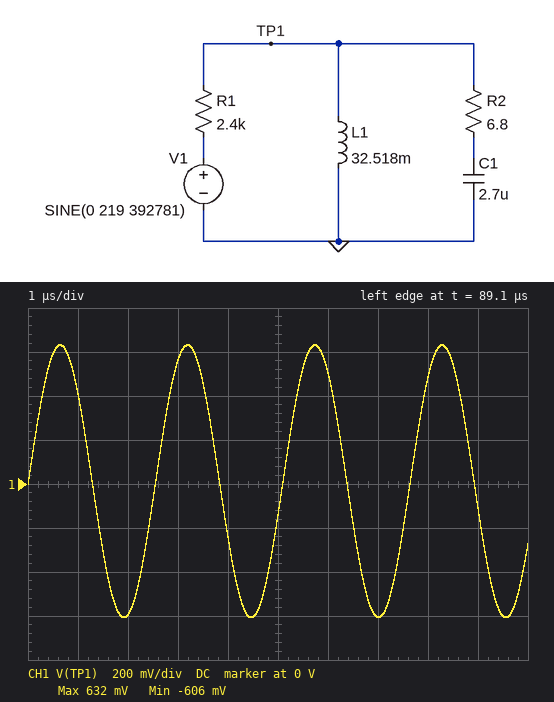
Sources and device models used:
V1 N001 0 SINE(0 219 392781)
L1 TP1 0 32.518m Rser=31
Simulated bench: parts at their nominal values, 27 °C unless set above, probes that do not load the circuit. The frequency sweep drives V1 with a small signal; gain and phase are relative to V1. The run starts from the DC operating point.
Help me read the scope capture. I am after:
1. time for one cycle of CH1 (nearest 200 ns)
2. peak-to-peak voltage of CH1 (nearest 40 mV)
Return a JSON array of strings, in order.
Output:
["2.6 µs", "1.24 V"]
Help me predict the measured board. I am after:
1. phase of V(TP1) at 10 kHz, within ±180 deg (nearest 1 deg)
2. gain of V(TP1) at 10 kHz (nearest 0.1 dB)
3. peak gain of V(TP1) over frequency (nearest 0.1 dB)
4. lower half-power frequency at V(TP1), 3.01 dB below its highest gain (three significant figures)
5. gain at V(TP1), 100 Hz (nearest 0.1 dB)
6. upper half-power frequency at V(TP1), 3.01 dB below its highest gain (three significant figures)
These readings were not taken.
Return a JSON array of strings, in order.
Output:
["-41 deg", "-48.5 dB", "-18.3 dB", "442 Hz", "-36.0 dB", "652 Hz"]
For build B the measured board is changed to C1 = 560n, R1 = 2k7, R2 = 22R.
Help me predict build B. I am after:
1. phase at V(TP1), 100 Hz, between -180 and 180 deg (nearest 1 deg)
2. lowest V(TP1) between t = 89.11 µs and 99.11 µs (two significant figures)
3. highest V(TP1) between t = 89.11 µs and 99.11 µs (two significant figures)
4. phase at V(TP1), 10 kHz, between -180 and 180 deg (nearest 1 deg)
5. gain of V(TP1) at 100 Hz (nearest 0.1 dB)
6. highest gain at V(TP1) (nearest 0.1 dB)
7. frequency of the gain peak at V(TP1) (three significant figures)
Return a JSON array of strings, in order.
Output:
["32 deg", "-1.7 V", "1.8 V", "-51 deg", "-37.3 dB", "-10.7 dB", "1.18 kHz"]
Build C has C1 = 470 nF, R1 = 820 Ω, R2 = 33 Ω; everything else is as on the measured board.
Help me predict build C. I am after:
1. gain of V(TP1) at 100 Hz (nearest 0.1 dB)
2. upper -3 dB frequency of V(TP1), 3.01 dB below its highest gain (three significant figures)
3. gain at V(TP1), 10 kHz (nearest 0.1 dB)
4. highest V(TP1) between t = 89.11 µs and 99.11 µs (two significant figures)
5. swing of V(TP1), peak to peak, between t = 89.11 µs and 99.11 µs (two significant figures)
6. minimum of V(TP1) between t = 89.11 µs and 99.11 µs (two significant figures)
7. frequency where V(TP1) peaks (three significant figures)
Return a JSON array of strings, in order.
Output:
["-27.2 dB", "1.69 kHz", "-25.0 dB", "8.6 V", "17 V", "-8.4 V", "1.29 kHz"]
